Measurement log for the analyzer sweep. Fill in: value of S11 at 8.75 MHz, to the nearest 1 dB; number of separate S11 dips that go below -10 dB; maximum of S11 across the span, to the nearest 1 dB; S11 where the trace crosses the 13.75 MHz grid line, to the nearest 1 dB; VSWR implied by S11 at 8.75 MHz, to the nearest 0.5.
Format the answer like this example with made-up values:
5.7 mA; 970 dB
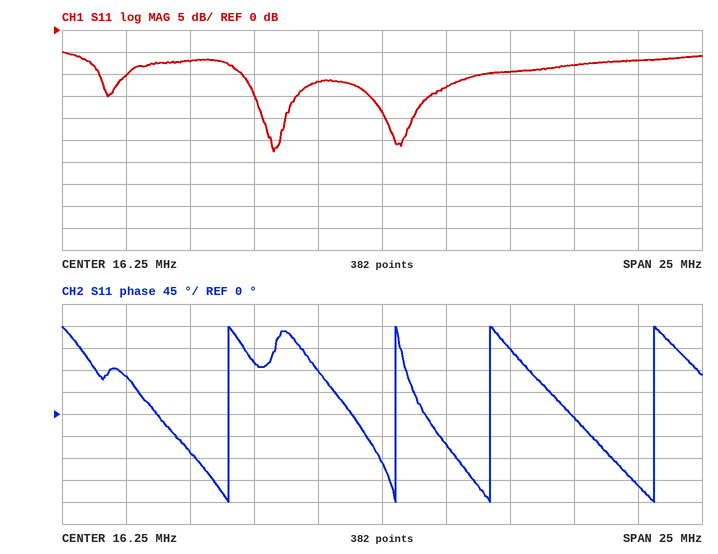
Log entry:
-7 dB; 3; -5 dB; -12 dB; 2.5
